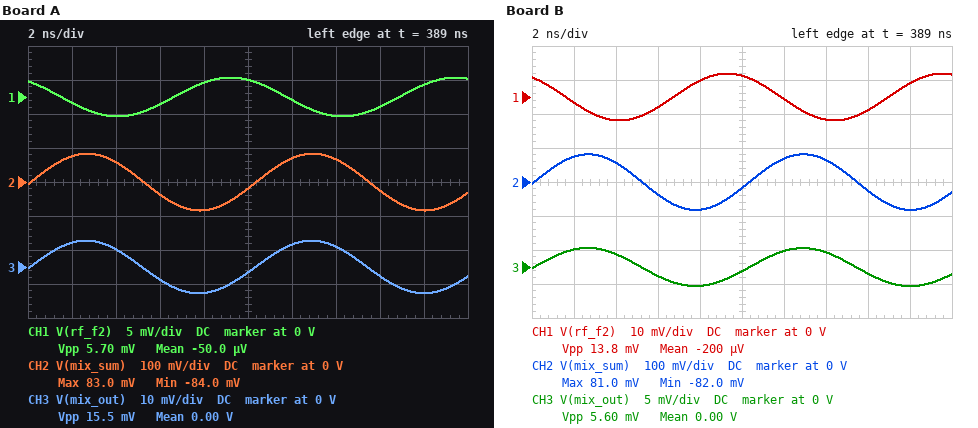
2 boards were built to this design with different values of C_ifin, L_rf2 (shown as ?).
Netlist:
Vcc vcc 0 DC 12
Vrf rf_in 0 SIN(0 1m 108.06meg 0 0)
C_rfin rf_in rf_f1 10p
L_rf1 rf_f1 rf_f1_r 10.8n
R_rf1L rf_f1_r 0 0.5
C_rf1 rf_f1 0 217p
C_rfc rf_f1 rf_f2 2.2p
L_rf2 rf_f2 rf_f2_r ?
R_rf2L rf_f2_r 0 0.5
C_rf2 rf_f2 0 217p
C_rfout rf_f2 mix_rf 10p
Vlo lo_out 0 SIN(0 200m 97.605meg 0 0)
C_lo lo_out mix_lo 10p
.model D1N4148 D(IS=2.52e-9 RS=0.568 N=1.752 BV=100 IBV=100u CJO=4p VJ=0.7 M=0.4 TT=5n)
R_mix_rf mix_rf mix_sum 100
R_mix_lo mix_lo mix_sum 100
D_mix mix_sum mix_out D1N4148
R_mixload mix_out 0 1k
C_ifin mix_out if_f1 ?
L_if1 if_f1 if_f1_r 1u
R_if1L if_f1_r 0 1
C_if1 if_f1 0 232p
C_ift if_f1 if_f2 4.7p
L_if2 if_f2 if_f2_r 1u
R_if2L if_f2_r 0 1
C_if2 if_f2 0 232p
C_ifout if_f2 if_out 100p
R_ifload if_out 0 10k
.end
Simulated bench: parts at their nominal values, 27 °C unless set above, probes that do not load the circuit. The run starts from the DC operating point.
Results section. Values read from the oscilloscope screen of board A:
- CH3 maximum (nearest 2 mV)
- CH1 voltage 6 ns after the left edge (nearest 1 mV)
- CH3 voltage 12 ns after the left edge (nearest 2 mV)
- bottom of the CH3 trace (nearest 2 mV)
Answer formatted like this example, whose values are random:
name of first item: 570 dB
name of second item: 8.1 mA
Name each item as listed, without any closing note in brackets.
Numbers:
CH3 maximum: 8 mV
CH1 voltage 6 ns after the left edge: -1 mV
CH3 voltage 12 ns after the left edge: 6 mV
bottom of the CH3 trace: -8 mV
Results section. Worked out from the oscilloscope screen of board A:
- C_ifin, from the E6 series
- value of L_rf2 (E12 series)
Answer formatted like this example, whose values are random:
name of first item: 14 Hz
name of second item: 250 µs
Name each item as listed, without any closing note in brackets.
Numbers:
C_ifin, from the E6 series: 47 pF
value of L_rf2: 5.6 nH
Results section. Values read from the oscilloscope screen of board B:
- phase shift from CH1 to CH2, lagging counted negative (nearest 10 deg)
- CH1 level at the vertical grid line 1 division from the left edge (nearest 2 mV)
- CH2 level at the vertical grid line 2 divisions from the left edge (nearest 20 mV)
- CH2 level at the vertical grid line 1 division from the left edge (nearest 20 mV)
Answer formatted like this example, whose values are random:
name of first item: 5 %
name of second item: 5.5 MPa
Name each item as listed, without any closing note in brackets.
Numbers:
phase shift from CH1 to CH2, lagging counted negative: -130 deg
CH1 level at the vertical grid line 1 division from the left edge: -2 mV
CH2 level at the vertical grid line 2 divisions from the left edge: 60 mV
CH2 level at the vertical grid line 1 division from the left edge: 80 mV
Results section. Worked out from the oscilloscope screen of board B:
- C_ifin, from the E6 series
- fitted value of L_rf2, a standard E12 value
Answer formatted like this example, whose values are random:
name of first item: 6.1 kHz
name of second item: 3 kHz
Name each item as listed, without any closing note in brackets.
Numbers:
C_ifin, from the E6 series: 220 pF
fitted value of L_rf2, a standard E12 value: 8.2 nH
